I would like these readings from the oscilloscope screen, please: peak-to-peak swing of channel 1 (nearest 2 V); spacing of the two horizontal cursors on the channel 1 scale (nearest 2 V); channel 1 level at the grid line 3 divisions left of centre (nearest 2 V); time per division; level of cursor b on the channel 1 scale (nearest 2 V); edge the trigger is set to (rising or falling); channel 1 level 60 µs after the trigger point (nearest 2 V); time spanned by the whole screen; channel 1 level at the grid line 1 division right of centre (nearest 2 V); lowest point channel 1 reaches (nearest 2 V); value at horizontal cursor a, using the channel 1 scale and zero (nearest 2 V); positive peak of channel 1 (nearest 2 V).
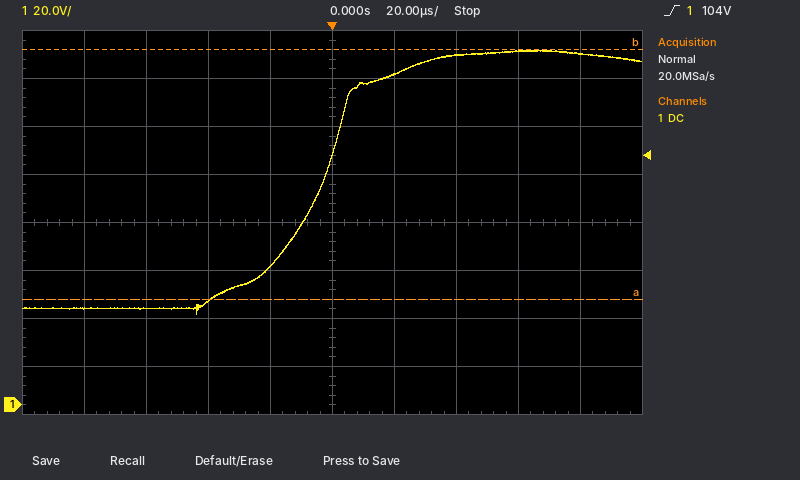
110 V
104 V
40 V
20 µs
148 V
rising
148 V
200 µs
138 V
38 V
44 V
148 V
